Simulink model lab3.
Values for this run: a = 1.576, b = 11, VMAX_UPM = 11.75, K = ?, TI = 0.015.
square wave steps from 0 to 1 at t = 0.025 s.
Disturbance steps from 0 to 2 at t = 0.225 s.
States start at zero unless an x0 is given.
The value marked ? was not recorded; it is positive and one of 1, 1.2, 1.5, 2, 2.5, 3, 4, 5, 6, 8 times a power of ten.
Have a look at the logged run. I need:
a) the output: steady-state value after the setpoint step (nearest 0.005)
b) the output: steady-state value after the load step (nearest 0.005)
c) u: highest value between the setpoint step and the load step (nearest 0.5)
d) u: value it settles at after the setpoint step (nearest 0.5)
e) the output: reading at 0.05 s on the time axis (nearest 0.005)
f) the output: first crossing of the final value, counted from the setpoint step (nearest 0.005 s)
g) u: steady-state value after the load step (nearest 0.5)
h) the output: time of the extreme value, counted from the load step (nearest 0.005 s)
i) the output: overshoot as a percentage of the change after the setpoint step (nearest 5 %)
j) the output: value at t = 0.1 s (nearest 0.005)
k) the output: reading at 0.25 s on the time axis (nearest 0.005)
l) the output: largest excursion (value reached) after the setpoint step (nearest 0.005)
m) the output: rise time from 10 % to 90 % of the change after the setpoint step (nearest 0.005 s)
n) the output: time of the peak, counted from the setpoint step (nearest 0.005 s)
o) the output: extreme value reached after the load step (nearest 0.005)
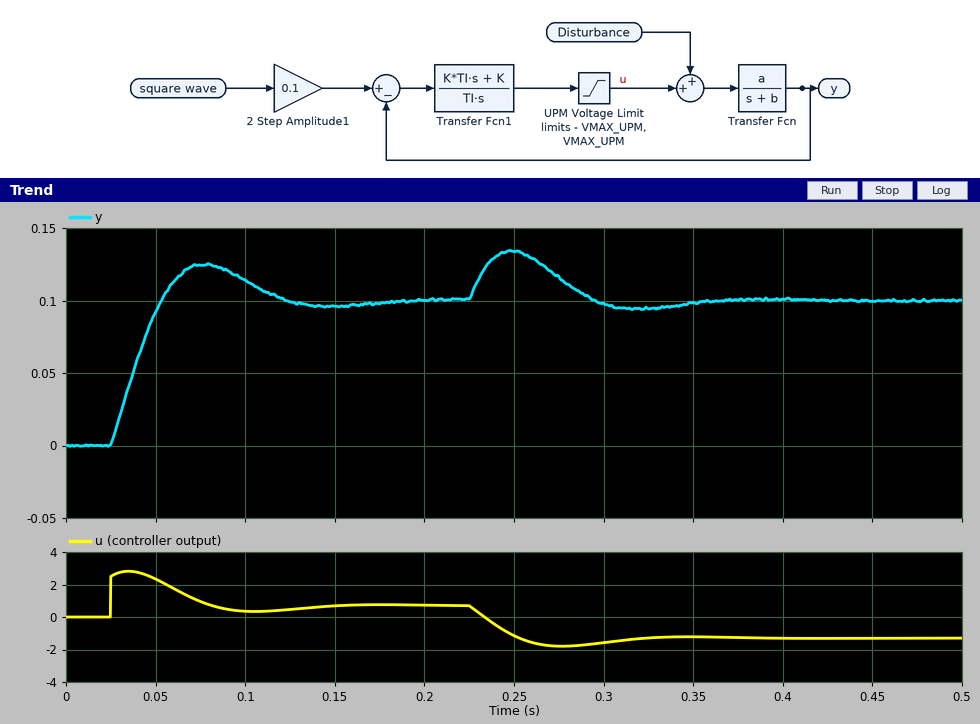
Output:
0.100
0.100
3.0
0.5
0.090
0.030 s
-1.5
0.025 s
25 %
0.115
0.135
0.125
0.020 s
0.050 s
0.135
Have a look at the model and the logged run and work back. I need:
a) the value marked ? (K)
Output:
25
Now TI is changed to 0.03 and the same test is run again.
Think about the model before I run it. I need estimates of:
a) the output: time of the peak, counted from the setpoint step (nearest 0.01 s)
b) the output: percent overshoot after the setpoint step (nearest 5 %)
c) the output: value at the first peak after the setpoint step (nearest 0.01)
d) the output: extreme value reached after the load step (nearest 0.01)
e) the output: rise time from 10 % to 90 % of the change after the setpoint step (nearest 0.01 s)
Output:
0.07 s
15 %
0.11
0.14
0.03 s
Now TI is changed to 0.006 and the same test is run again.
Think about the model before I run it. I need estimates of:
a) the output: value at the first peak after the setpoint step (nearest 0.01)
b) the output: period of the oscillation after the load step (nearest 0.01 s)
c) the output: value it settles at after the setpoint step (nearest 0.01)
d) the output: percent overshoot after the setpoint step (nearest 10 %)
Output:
0.14
0.08 s
0.10
40 %
